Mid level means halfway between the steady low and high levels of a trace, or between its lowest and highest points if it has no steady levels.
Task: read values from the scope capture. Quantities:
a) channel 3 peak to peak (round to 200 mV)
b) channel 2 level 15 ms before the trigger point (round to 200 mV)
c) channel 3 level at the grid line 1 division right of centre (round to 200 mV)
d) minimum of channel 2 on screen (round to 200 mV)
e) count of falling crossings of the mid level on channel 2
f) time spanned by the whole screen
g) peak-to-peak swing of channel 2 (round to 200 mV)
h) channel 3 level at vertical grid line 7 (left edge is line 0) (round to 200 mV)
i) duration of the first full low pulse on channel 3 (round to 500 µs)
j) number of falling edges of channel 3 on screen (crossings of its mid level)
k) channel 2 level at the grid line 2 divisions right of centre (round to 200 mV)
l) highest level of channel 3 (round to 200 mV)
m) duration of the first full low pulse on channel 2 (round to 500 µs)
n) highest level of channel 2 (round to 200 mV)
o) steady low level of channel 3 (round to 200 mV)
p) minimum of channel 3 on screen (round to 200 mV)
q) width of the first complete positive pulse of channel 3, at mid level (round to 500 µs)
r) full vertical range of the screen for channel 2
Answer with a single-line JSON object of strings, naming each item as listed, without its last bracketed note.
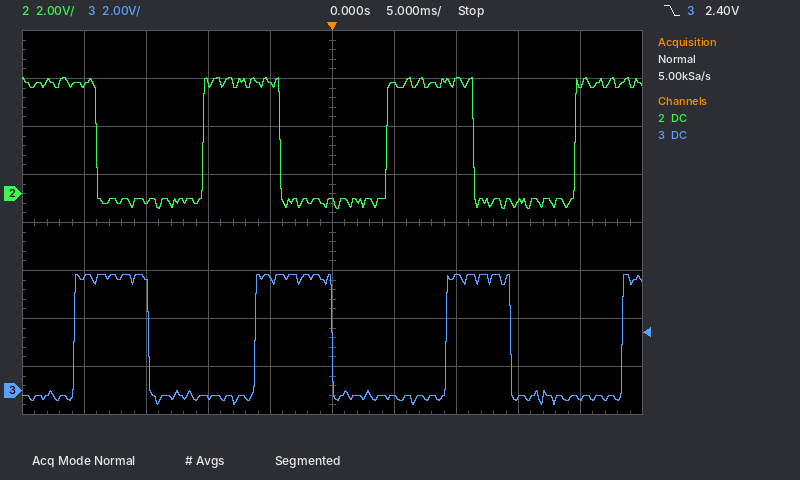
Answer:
{"channel 3 peak to peak": "5.4 V", "channel 2 level 15 ms before the trigger point": "-400 mV", "channel 3 level at the grid line 1 division right of centre": "-200 mV", "minimum of channel 2 on screen": "-600 mV", "count of falling crossings of the mid level on channel 2": "3", "time spanned by the whole screen": "50 ms", "peak-to-peak swing of channel 2": "5.4 V", "channel 3 level at vertical grid line 7 (left edge is line 0)": "4.8 V", "duration of the first full low pulse on channel 3": "8.5 ms", "number of falling edges of channel 3 on screen": "3", "channel 2 level at the grid line 2 divisions right of centre": "4.6 V", "highest level of channel 3": "4.8 V", "duration of the first full low pulse on channel 2": "8.5 ms", "highest level of channel 2": "4.8 V", "steady low level of channel 3": "-200 mV", "minimum of channel 3 on screen": "-600 mV", "width of the first complete positive pulse of channel 3, at mid level": "6.0 ms", "full vertical range of the screen for channel 2": "16 V"}
